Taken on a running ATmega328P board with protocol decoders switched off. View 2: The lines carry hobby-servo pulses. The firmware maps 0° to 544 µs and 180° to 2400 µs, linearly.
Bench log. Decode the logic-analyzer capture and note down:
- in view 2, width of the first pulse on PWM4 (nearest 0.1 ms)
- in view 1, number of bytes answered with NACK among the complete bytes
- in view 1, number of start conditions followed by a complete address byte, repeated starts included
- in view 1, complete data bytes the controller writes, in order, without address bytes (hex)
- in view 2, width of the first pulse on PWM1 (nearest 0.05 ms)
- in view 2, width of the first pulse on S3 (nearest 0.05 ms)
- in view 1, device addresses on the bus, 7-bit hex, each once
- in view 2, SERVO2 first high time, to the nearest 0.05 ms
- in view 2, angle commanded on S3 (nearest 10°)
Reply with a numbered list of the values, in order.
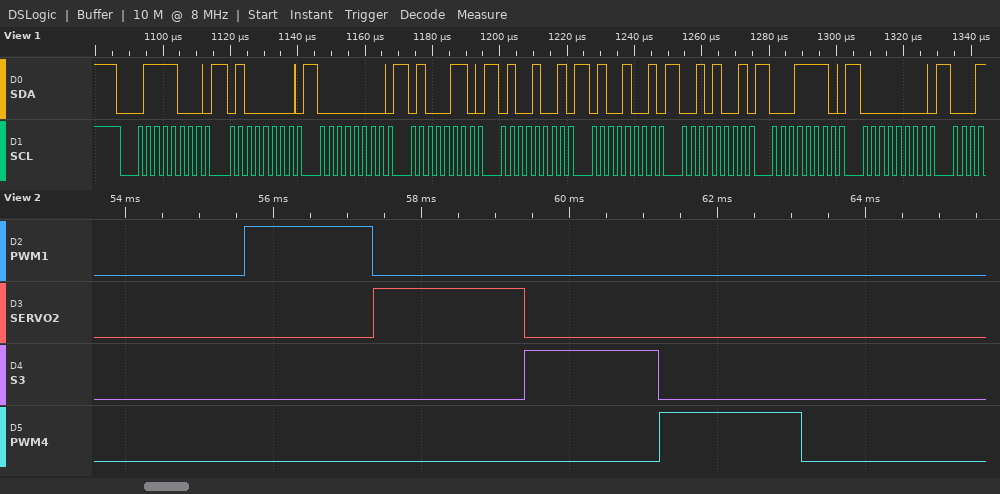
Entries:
1. 1.9 ms
2. 0
3. 1
4. 40 00 46 49 49 29 1E 00
5. 1.75 ms
6. 1.80 ms
7. 0x3C
8. 2.05 ms
9. 120°
